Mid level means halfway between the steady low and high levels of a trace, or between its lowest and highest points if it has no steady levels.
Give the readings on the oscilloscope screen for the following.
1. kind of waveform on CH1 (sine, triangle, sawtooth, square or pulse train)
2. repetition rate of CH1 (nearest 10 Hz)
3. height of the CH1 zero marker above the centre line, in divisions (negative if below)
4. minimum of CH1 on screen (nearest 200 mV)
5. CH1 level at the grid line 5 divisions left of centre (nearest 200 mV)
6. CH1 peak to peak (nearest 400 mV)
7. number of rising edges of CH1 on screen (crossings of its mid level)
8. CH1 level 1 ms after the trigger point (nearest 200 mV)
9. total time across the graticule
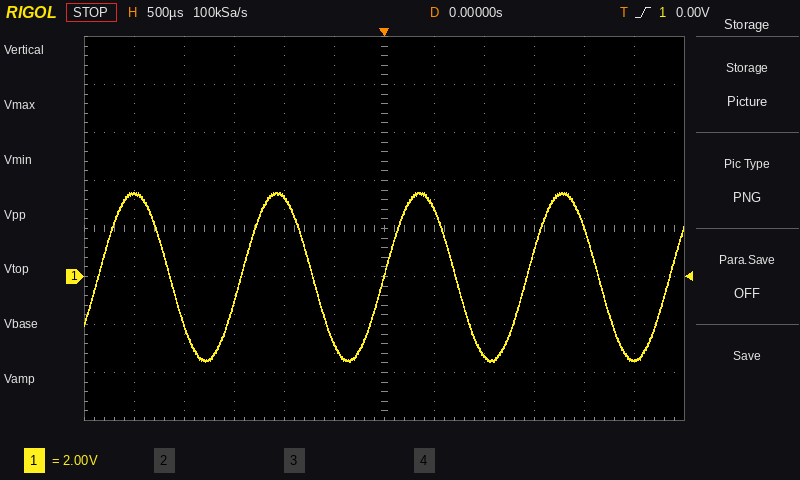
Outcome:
sine
700 Hz
-1.0 div
-3.6 V
3.4 V
7.2 V
5
-3.2 V
6 ms
